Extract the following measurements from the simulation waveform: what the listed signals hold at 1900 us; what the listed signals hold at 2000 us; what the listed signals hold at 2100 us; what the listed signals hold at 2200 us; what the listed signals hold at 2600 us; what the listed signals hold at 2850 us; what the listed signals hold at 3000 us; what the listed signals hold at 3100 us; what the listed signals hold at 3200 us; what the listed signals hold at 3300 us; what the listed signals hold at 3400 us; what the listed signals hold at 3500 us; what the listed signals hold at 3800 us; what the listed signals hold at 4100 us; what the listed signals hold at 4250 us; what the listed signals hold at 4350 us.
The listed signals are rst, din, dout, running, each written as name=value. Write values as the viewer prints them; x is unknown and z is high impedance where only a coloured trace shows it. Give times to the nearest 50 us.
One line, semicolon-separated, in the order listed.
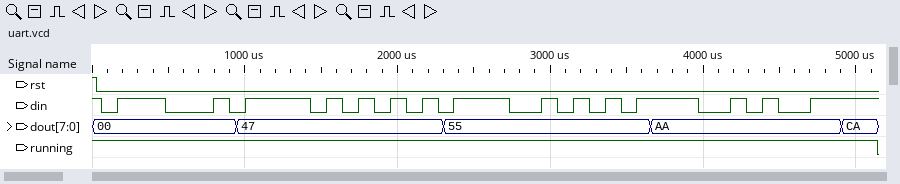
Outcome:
rst=0, din=0, dout=47, running=1; rst=0, din=1, dout=47, running=1; rst=0, din=0, dout=47, running=1; rst=0, din=1, dout=47, running=1; rst=0, din=1, dout=55, running=1; rst=0, din=0, dout=55, running=1; rst=0, din=1, dout=55, running=1; rst=0, din=0, dout=55, running=1; rst=0, din=1, dout=55, running=1; rst=0, din=0, dout=55, running=1; rst=0, din=1, dout=55, running=1; rst=0, din=0, dout=55, running=1; rst=0, din=1, dout=AA, running=1; rst=0, din=0, dout=AA, running=1; rst=0, din=1, dout=AA, running=1; rst=0, din=0, dout=AA, running=1
